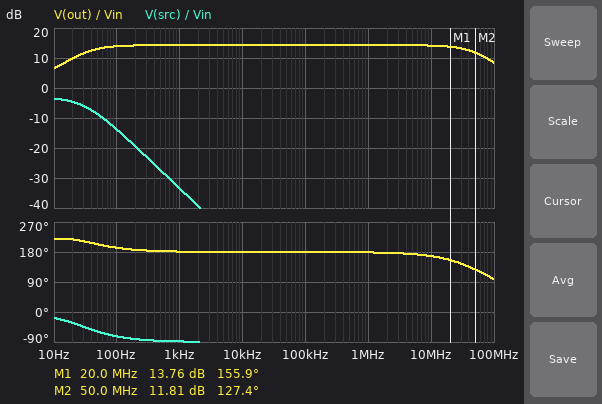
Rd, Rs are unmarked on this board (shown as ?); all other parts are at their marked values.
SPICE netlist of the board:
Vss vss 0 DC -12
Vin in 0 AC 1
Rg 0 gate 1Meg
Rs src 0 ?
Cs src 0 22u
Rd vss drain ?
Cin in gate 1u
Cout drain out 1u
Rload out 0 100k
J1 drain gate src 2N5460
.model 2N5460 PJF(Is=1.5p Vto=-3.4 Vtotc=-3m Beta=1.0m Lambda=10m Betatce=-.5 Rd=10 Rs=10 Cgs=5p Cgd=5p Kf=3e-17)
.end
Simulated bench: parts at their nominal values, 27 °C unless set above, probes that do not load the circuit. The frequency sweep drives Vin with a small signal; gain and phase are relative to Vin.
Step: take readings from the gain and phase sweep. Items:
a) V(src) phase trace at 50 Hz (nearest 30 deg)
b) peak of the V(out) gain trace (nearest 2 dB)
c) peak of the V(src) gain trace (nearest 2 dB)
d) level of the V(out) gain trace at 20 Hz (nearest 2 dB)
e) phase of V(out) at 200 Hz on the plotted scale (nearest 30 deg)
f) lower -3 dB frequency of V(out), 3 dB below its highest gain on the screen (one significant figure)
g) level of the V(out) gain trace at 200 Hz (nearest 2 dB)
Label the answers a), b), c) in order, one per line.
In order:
a) -60 deg
b) 14 dB
c) -4 dB
d) 10 dB
e) 180 deg
f) 30 Hz
g) 14 dB
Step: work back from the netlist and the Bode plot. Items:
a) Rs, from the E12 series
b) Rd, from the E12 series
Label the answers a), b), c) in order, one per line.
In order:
a) 820 Ω
b) 1.8 kΩ
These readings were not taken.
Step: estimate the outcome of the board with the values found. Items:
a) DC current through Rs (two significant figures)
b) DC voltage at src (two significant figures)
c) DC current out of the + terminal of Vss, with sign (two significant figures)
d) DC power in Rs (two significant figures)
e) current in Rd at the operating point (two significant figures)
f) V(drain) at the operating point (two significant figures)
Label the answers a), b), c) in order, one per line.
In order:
a) 2.3 mA
b) -1.9 V
c) -2.3 mA
d) 4.4 mW
e) 2.3 mA
f) -7.8 V
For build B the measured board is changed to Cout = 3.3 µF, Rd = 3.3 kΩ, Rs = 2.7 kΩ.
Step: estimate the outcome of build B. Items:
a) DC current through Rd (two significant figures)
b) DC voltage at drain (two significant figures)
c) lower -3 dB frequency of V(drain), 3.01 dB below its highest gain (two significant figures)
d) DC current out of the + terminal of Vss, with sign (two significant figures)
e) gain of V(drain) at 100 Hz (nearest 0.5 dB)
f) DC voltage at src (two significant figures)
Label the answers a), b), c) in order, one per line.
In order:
a) 910 µA
b) -9.0 V
c) 16 Hz
d) -910 µA
e) 15.5 dB
f) -2.5 V
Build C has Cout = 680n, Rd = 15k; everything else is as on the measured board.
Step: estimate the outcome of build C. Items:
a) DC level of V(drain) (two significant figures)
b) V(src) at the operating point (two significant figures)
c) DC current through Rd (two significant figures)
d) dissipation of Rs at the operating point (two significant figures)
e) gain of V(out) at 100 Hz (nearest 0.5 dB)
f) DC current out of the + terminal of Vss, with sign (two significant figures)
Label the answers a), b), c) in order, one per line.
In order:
a) -770 mV
b) -610 mV
c) 750 µA
d) 460 µW
e) -26.0 dB
f) -750 µA
